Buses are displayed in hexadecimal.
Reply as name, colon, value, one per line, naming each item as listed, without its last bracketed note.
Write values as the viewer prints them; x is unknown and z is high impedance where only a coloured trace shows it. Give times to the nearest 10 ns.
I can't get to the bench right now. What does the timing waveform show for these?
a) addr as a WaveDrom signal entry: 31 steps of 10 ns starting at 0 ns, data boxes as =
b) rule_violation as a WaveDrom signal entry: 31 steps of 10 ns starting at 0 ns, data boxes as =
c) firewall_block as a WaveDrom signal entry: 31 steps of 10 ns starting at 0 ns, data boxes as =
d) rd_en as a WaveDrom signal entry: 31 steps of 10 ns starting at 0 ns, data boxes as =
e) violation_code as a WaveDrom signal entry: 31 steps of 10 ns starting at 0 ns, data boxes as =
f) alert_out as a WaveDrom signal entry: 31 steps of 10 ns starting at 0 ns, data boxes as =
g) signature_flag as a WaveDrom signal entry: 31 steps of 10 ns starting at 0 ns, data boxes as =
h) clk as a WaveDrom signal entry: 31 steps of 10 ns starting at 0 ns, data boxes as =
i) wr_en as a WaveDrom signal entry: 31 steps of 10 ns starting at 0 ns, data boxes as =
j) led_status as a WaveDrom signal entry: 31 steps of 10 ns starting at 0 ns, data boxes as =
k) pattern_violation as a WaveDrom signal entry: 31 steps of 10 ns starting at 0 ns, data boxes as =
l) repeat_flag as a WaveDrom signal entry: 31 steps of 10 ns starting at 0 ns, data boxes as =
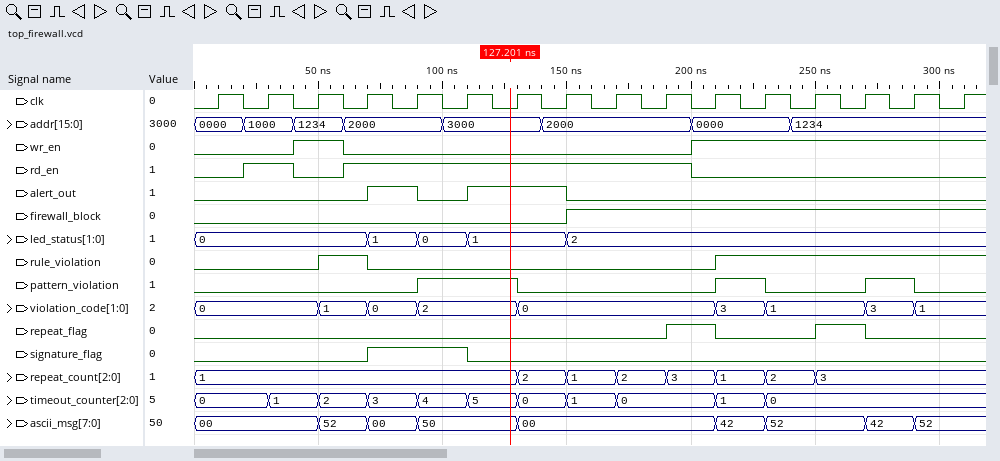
addr as a WaveDrom signal entry: 31 steps of 10 ns starting at 0 ns, data boxes as =: {name: 'addr', wave: '=.=.=.=...=...=.....=...=......', data: '0000 1000 1234 2000 3000 2000 0000 1234'}
rule_violation as a WaveDrom signal entry: 31 steps of 10 ns starting at 0 ns, data boxes as =: {name: 'rule_violation', wave: '0....1.0.............1.........'}
firewall_block as a WaveDrom signal entry: 31 steps of 10 ns starting at 0 ns, data boxes as =: {name: 'firewall_block', wave: '0..............1...............'}
rd_en as a WaveDrom signal entry: 31 steps of 10 ns starting at 0 ns, data boxes as =: {name: 'rd_en', wave: '0.1.0.1.............0..........'}
violation_code as a WaveDrom signal entry: 31 steps of 10 ns starting at 0 ns, data boxes as =: {name: 'violation_code', wave: '=....=.=.=...=.......=.=...=.=.', data: '0 1 0 2 0 3 1 3 1'}
alert_out as a WaveDrom signal entry: 31 steps of 10 ns starting at 0 ns, data boxes as =: {name: 'alert_out', wave: '0......1.0.1...0...............'}
signature_flag as a WaveDrom signal entry: 31 steps of 10 ns starting at 0 ns, data boxes as =: {name: 'signature_flag', wave: '0......1...0...................'}
clk as a WaveDrom signal entry: 31 steps of 10 ns starting at 0 ns, data boxes as =: {name: 'clk', wave: '0101010101010101010101010101010'}
wr_en as a WaveDrom signal entry: 31 steps of 10 ns starting at 0 ns, data boxes as =: {name: 'wr_en', wave: '0...1.0.............1..........'}
led_status as a WaveDrom signal entry: 31 steps of 10 ns starting at 0 ns, data boxes as =: {name: 'led_status', wave: '=......=.=.=...=...............', data: '0 1 0 1 2'}
pattern_violation as a WaveDrom signal entry: 31 steps of 10 ns starting at 0 ns, data boxes as =: {name: 'pattern_violation', wave: '0........1...0.......1.0...1.0.'}
repeat_flag as a WaveDrom signal entry: 31 steps of 10 ns starting at 0 ns, data boxes as =: {name: 'repeat_flag', wave: '0..................1.0...1.0...'}
